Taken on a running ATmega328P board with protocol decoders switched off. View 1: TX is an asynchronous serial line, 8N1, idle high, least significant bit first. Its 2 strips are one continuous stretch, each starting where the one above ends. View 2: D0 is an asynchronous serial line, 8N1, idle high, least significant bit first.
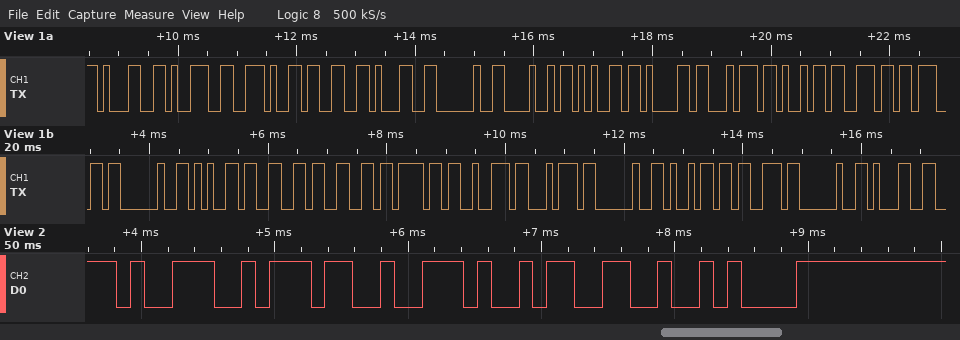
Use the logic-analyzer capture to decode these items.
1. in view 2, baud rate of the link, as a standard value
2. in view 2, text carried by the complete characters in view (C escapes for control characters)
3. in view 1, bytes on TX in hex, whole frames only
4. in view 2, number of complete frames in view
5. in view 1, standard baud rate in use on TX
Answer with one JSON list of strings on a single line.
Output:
["9600 baud", "\"97.3\\n\"", "0x31 0x39 0x2E 0x33 0x31 0x20 0x48 0x65 0x61 0x74 0x69 0x6E 0x67 0x20 0x65 0x66 0x66 0x6F 0x72 0x74 0x20 0x69 0x73 0x20 0x31", "5", "9600 baud"]
